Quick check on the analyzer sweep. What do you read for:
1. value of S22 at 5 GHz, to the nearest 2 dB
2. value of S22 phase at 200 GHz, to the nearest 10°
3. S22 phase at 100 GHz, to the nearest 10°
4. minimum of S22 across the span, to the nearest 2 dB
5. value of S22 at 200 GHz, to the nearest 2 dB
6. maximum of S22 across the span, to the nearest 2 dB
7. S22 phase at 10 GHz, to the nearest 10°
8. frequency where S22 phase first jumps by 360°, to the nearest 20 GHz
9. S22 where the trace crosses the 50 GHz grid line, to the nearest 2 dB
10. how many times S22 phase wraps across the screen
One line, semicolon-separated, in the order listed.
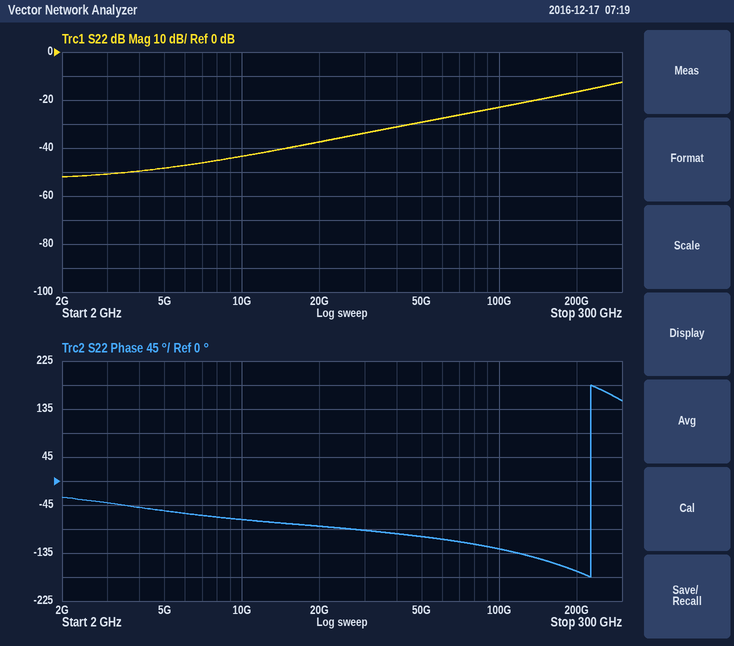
-48 dB; -170°; -130°; -52 dB; -16 dB; -12 dB; -70°; 220 GHz; -30 dB; 1
